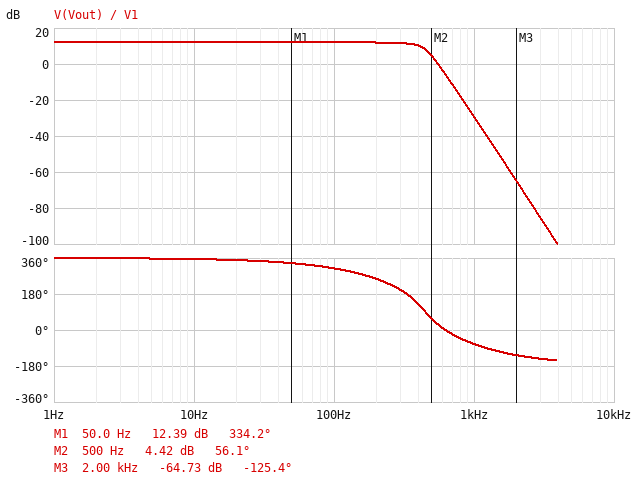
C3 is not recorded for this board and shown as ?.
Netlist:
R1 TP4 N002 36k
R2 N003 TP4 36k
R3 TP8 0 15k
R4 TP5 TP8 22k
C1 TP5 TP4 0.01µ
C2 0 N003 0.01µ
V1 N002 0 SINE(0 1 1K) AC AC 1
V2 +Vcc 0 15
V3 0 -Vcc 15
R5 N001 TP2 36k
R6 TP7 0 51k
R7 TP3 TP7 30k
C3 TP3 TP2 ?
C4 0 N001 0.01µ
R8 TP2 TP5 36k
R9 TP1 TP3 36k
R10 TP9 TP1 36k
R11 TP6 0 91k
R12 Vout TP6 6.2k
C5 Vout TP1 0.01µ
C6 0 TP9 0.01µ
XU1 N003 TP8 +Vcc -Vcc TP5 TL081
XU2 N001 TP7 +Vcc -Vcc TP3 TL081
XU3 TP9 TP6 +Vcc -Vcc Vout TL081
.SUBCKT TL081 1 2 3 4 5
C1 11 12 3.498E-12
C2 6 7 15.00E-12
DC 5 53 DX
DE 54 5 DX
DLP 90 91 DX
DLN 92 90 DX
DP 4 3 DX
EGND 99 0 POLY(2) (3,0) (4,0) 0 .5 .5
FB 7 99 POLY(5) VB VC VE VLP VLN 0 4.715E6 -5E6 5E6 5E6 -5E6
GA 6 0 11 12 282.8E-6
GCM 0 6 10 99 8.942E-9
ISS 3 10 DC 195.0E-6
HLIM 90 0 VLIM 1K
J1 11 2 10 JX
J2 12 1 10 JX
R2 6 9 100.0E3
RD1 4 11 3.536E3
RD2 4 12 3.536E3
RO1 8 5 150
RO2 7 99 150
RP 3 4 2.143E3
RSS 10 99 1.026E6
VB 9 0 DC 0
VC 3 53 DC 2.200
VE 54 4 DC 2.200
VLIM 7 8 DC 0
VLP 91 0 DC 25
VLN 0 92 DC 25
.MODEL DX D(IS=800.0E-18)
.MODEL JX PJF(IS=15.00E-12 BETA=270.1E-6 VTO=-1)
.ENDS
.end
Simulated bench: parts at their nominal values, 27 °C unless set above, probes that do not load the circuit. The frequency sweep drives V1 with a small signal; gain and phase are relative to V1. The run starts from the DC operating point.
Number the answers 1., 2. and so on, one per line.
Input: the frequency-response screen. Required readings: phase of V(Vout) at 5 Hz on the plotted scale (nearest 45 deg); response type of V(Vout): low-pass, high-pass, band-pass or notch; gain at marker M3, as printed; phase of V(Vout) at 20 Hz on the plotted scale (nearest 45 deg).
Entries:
1. 360 deg
2. low-pass
3. -64.73 dB
4. 360 deg
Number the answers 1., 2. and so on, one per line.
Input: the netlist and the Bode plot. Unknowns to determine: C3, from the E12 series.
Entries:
1. 8.2 nF
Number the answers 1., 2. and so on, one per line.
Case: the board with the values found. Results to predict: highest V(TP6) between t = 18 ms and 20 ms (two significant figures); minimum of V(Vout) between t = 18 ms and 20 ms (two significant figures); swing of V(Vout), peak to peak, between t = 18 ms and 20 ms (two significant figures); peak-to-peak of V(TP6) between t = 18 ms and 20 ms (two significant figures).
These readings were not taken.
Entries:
1. 32 mV
2. -35 mV
3. 69 mV
4. 65 mV
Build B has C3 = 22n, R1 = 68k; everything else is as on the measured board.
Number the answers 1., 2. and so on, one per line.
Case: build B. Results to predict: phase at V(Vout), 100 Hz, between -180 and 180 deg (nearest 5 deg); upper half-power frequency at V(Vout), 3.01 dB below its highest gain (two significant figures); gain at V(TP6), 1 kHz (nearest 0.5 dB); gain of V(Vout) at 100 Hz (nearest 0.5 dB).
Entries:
1. -35 deg
2. 330 Hz
3. -43.0 dB
4. 14.0 dB
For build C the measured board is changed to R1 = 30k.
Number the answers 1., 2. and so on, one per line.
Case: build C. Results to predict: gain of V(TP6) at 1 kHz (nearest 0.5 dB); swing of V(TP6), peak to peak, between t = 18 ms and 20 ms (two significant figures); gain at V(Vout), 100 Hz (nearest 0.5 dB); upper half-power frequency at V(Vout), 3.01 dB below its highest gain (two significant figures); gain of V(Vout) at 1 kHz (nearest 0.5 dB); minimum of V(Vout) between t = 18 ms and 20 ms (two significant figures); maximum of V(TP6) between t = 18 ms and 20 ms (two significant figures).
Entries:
1. -28.0 dB
2. 78 mV
3. 12.0 dB
4. 360 Hz
5. -27.5 dB
6. -42 mV
7. 39 mV
